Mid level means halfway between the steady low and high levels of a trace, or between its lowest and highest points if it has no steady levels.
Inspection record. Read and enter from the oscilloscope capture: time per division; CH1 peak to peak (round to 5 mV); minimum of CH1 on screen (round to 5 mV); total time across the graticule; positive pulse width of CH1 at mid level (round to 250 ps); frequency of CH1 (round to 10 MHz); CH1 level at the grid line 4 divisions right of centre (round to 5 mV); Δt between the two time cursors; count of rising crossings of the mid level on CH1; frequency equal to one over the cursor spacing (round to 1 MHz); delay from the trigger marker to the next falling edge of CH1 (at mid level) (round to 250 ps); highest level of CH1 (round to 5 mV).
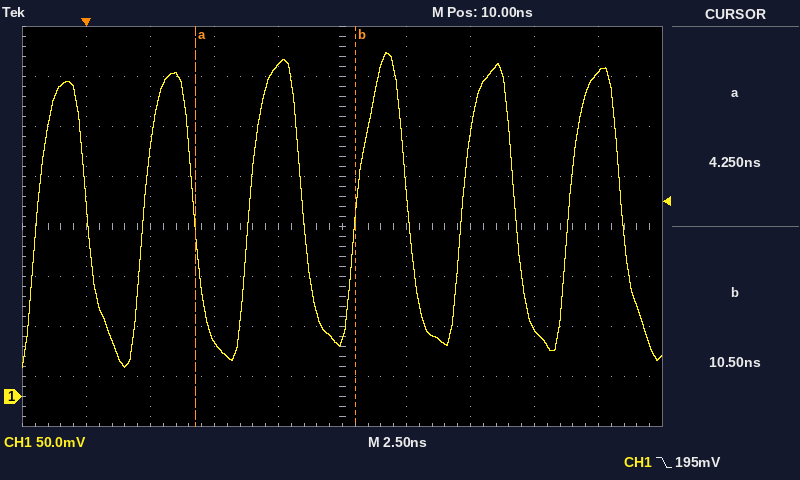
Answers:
2.5 ns
315 mV
30 mV
25 ns
2.00 ns
240 MHz
325 mV
6.25 ns
6
160 MHz
4.25 ns
345 mV
